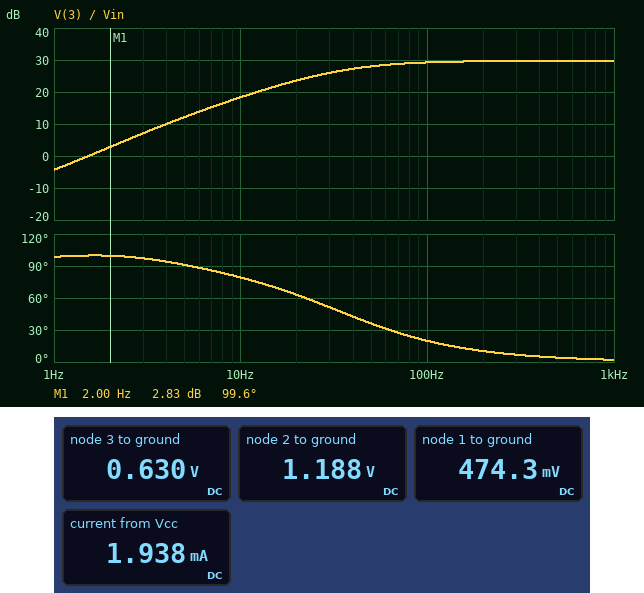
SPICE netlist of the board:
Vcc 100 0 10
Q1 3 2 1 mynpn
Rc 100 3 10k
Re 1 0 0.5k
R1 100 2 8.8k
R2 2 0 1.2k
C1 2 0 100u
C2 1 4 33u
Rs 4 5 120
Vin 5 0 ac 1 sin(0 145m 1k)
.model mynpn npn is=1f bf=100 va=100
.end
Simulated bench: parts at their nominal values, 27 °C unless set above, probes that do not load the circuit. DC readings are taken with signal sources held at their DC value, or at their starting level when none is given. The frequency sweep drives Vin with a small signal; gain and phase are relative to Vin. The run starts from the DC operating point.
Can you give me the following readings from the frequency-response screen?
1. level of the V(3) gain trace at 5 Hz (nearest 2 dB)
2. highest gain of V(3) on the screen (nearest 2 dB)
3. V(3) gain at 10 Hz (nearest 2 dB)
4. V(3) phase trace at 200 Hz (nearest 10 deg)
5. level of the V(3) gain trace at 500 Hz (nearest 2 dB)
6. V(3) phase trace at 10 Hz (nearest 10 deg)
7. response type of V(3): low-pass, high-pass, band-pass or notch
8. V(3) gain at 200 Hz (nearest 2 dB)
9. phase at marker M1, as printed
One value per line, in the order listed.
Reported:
12 dB
30 dB
18 dB
10 deg
30 dB
80 deg
high-pass
30 dB
99.6 deg
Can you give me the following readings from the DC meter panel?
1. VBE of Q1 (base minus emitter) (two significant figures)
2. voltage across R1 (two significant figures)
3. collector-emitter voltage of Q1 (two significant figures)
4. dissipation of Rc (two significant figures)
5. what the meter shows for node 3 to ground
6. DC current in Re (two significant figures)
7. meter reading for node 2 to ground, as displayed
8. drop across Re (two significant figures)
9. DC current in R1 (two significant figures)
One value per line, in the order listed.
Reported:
710 mV
8.8 V
160 mV
8.8 mW
0.630 V
950 µA
1.188 V
470 mV
1.0 mA
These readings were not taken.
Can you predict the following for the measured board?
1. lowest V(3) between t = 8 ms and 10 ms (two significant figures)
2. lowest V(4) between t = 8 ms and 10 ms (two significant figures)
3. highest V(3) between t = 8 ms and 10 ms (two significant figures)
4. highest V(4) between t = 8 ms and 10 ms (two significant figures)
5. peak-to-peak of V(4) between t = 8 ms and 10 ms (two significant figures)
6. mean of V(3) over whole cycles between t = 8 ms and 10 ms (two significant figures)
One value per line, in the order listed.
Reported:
460 mV
-39 mV
8.7 V
40 mV
79 mV
3.5 V
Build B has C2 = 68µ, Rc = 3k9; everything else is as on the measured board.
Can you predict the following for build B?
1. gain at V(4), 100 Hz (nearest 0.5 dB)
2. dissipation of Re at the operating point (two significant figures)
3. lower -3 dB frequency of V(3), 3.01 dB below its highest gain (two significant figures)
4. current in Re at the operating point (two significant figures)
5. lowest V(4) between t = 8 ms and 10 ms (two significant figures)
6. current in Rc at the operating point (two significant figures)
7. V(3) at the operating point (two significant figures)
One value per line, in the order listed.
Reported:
-12.5 dB
460 µW
16 Hz
960 µA
-23 mV
950 µA
6.3 V
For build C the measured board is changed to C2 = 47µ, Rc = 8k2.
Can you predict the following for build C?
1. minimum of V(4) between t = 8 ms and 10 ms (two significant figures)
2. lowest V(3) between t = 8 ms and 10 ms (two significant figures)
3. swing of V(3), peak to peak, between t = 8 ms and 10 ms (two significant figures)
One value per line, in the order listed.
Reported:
-36 mV
470 mV
8.4 V
